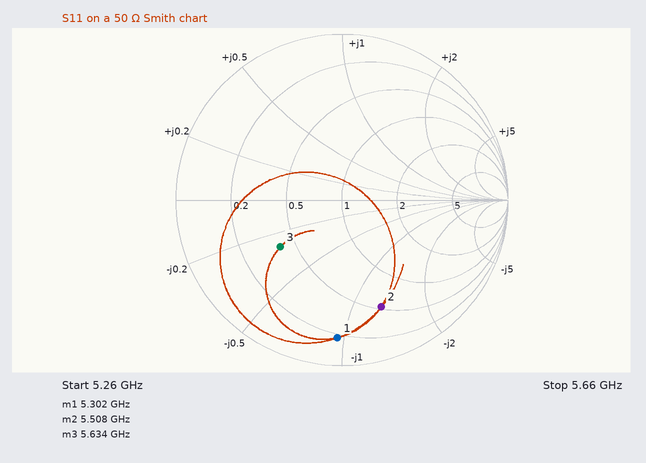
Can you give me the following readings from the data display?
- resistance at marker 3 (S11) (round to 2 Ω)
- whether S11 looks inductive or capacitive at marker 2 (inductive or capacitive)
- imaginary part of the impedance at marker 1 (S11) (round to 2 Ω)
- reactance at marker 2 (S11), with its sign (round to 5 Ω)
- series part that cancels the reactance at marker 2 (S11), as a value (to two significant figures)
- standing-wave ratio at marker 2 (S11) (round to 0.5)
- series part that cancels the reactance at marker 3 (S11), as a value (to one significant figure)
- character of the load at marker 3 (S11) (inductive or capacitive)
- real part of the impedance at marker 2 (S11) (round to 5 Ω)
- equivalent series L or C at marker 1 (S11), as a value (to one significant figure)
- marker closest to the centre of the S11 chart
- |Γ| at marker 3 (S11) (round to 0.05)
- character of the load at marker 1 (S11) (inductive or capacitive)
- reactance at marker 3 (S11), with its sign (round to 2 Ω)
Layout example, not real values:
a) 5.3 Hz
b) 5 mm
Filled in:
a) 20 Ω
b) capacitive
c) -48 Ω
d) -65 Ω
e) 1.9 nH
f) 5.5
g) 400 pH
h) capacitive
i) 25 Ω
j) 600 fF
k) marker 3
l) 0.45
m) capacitive
n) -14 Ω
